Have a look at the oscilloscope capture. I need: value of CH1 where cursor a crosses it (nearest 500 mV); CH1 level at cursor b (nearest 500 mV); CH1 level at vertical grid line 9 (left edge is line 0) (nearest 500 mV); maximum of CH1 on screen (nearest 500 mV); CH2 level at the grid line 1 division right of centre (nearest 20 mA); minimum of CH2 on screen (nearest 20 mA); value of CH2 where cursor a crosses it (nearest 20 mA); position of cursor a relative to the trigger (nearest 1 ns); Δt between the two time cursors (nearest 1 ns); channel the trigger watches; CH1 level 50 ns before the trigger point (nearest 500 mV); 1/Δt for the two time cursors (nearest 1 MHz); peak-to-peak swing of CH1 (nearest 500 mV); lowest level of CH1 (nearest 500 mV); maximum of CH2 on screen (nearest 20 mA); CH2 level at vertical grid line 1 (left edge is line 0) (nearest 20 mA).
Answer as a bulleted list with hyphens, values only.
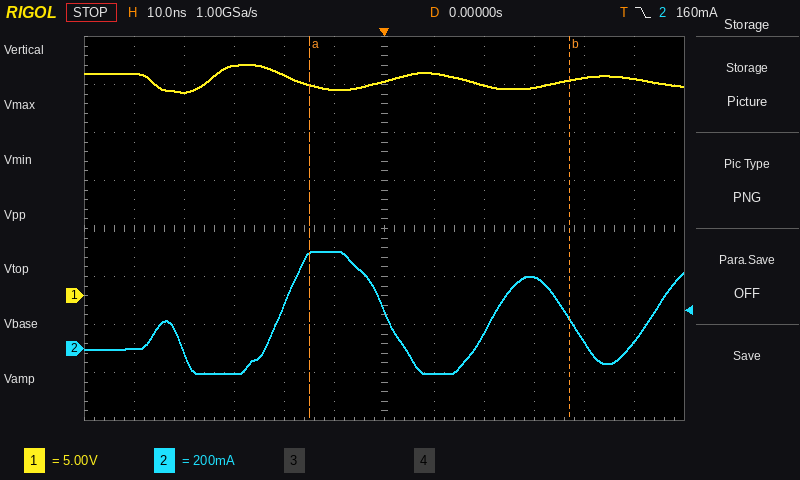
- 22.0 V
- 22.5 V
- 21.5 V
- 24.0 V
- -100 mA
- -100 mA
- 400 mA
- -15 ns
- 52 ns
- CH2
- 23.0 V
- 19 MHz
- 3.0 V
- 21.0 V
- 400 mA
- 0 mA
